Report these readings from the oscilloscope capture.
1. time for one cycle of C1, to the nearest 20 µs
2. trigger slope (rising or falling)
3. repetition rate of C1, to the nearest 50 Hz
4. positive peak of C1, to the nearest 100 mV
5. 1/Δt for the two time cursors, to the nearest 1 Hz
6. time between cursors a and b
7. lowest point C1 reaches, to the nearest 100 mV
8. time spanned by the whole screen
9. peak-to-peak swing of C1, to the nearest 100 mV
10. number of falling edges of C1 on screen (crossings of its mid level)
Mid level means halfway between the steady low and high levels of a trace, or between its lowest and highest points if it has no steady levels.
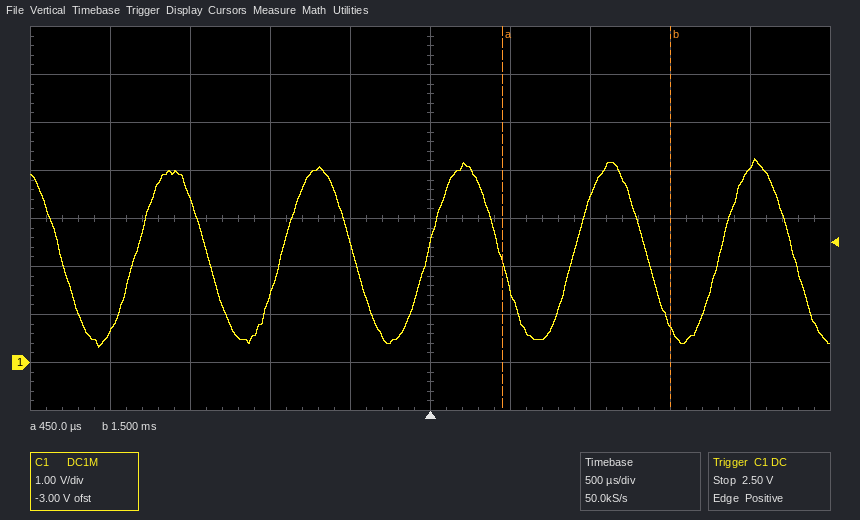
920 µs
rising
1.10 kHz
4.2 V
952 Hz
1.05 ms
300 mV
5 ms
3.9 V
6
